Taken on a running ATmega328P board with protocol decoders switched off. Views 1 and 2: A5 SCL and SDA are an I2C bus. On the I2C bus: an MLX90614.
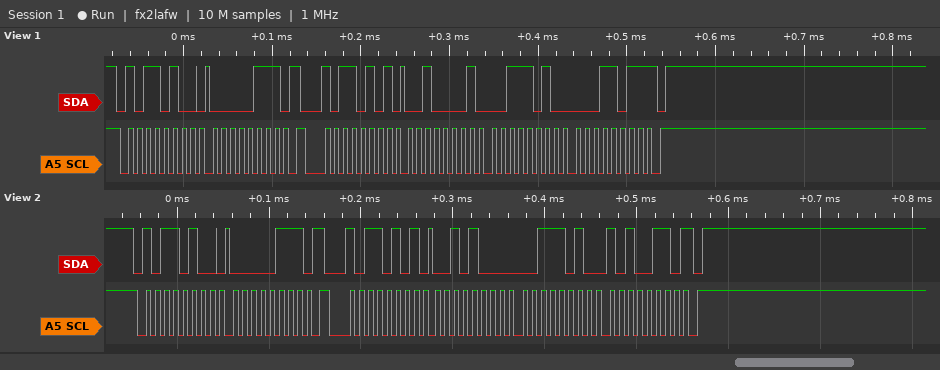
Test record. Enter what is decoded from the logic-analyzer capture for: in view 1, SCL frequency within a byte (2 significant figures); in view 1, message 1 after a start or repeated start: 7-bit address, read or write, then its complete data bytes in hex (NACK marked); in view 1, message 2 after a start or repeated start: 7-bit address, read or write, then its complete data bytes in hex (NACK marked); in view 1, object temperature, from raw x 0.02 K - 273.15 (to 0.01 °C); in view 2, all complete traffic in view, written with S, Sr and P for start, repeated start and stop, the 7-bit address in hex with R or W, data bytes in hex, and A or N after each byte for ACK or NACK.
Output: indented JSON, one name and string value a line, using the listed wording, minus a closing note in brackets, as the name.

{
  "in view 1, SCL frequency within a byte": "100 kHz",
  "in view 1, message 1 after a start or repeated start: 7-bit address, read or write, then its complete data bytes in hex": "0x5A write: 07",
  "in view 1, message 2 after a start or repeated start: 7-bit address, read or write, then its complete data bytes in hex": "0x5A read: 21 3A 1B NACK",
  "in view 1, object temperature, from raw x 0.02 K - 273.15": "24.47 °C",
  "in view 2, all complete traffic in view, written with S, Sr and P for start, repeated start and stop, the 7-bit address in hex with R or W, data bytes in hex, and A or N after each byte for ACK or NACK": "S 5AW A 07 A Sr 5AR A 28 A 3A A A6 N P"
}
